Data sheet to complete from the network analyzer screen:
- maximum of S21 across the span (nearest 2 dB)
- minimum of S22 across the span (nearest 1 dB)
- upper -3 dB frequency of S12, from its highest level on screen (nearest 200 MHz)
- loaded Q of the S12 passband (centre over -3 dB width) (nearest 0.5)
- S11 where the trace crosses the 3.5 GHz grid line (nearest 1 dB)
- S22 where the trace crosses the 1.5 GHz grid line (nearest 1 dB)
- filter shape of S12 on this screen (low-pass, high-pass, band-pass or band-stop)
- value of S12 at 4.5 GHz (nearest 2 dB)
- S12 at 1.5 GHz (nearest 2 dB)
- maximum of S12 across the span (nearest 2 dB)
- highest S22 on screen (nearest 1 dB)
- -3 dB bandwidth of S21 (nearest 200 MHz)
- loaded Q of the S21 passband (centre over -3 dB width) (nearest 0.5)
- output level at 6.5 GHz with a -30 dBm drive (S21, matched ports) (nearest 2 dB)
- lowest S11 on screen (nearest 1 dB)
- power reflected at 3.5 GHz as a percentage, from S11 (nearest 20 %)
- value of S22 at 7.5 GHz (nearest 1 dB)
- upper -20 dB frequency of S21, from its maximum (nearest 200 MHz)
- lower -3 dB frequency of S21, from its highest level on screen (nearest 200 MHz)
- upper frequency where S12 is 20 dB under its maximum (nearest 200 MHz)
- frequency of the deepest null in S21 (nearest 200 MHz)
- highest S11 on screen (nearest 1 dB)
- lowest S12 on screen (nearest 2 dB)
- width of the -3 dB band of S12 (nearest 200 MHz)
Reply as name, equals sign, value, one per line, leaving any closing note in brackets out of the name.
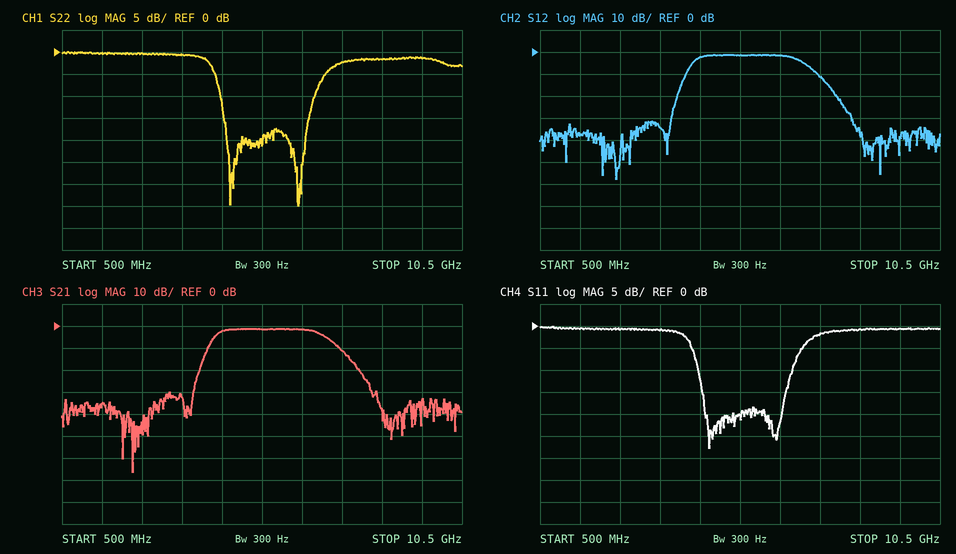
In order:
maximum of S21 across the span = -2 dB
minimum of S22 across the span = -35 dB
upper -3 dB frequency of S12, from its highest level on screen = 7.0 GHz
loaded Q of the S12 passband (centre over -3 dB width) = 2.0
S11 where the trace crosses the 3.5 GHz grid line = -1 dB
S22 where the trace crosses the 1.5 GHz grid line = 0 dB
filter shape of S12 on this screen = band-pass
value of S12 at 4.5 GHz = -2 dB
S12 at 1.5 GHz = -38 dB
maximum of S12 across the span = -2 dB
highest S22 on screen = 0 dB
-3 dB bandwidth of S21 = 2.6 GHz
loaded Q of the S21 passband (centre over -3 dB width) = 2.0
output level at 6.5 GHz with a -30 dBm drive (S21, matched ports) = -32 dBm
lowest S11 on screen = -28 dB
power reflected at 3.5 GHz as a percentage, from S11 = 80 %
value of S22 at 7.5 GHz = -2 dB
upper -20 dB frequency of S21, from its maximum = 8.0 GHz
lower -3 dB frequency of S21, from its highest level on screen = 4.4 GHz
upper frequency where S12 is 20 dB under its maximum = 8.0 GHz
frequency of the deepest null in S21 = 2.2 GHz
highest S11 on screen = 0 dB
lowest S12 on screen = -58 dB
width of the -3 dB band of S12 = 2.6 GHz
